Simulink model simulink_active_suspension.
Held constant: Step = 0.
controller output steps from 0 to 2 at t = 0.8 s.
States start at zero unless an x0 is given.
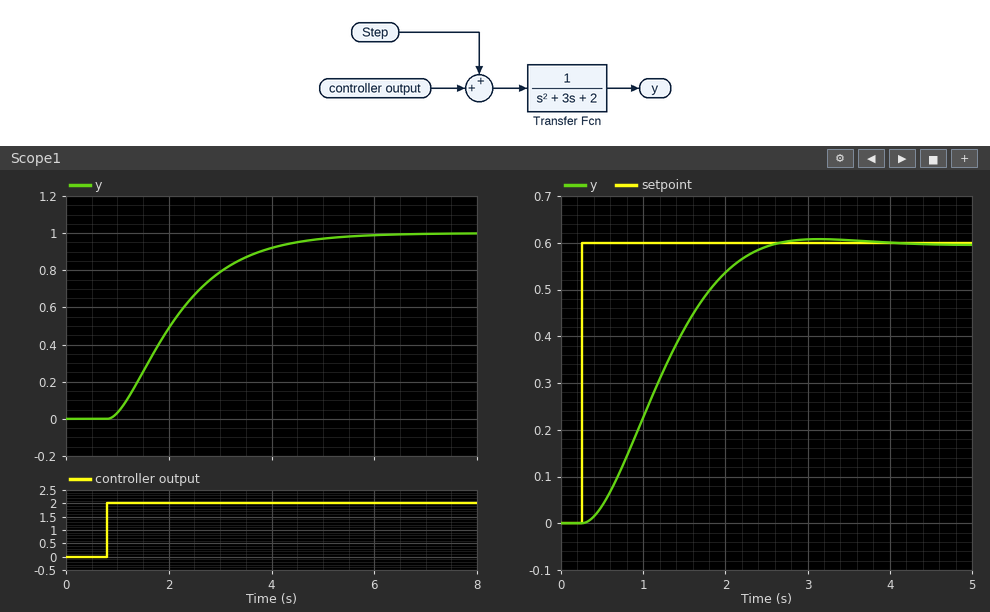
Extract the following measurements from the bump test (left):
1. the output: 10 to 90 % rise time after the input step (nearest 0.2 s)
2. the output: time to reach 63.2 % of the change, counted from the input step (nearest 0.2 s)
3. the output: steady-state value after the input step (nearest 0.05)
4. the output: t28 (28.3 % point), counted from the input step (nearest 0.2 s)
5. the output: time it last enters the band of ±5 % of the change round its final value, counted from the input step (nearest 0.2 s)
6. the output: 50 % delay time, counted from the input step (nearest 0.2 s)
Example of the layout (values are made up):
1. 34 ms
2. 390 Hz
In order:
1. 2.6 s
2. 1.6 s
3. 1.00
4. 0.8 s
5. 3.6 s
6. 1.2 s
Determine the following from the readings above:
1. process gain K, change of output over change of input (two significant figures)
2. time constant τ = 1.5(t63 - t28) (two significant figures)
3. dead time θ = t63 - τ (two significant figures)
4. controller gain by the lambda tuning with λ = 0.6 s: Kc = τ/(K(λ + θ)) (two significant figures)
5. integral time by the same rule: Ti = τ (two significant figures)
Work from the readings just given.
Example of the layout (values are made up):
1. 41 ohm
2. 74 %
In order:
1. 0.50
2. 1.2 s
3. 0.40 s
4. 2.4
5. 1.2 s
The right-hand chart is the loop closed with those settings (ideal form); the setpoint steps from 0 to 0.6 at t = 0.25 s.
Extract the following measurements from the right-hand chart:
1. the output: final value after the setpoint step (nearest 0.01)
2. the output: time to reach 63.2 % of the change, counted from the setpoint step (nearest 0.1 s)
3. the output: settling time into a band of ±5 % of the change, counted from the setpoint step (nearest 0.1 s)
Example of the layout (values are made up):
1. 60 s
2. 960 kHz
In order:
1. 0.60
2. 1.1 s
3. 2.0 s
